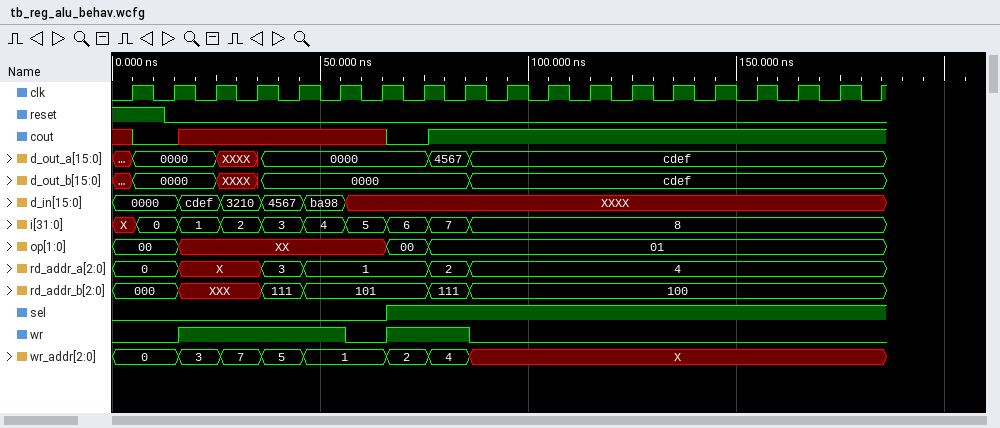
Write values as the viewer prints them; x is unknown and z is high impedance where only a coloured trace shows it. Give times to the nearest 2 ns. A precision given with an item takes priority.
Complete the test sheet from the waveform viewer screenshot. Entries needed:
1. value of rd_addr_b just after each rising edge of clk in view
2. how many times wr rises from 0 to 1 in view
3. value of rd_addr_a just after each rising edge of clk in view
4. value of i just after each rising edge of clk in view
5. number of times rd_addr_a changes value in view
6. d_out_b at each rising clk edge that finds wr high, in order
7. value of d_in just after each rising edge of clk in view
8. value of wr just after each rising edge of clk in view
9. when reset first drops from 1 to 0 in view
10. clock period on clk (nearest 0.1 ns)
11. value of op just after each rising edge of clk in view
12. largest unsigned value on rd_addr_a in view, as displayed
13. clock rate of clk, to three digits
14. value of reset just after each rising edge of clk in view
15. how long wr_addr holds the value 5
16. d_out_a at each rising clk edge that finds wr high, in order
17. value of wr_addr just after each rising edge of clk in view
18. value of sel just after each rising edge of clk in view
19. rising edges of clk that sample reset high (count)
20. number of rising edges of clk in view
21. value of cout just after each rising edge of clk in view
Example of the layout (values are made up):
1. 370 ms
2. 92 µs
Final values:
1. 000, 000, XXX, XXX, 111, 101, 101, 101, 111, 100, 100, 100, 100, 100, 100, 100, 100, 100, 100
2. 2
3. 0, 0, X, X, 3, 1, 1, 1, 2, 4, 4, 4, 4, 4, 4, 4, 4, 4, 4
4. X, 0, 1, 2, 3, 4, 5, 6, 7, 8, 8, 8, 8, 8, 8, 8, 8, 8, 8
5. 5
6. 0000, XXXX, 0000, 0000, 0000, 0000
7. 0000, 0000, cdef, 3210, 4567, ba98, XXXX, XXXX, XXXX, XXXX, XXXX, XXXX, XXXX, XXXX, XXXX, XXXX, XXXX, XXXX, XXXX
8. 0 0 1 1 1 1 0 1 1 0 0 0 0 0 0 0 0 0 0
9. 12 ns
10. 10 ns
11. 00, 00, XX, XX, XX, XX, XX, 00, 01, 01, 01, 01, 01, 01, 01, 01, 01, 01, 01
12. 4
13. 100 MHz
14. 1 0 0 0 0 0 0 0 0 0 0 0 0 0 0 0 0 0 0
15. 10 ns
16. 0000, XXXX, 0000, 0000, 0000, 4567
17. 0, 0, 3, 7, 5, 1, 1, 2, 4, X, X, X, X, X, X, X, X, X, X
18. 0 0 0 0 0 0 0 1 1 1 1 1 1 1 1 1 1 1 1
19. 1
20. 19
21. 0 0 x x x x x 0 1 1 1 1 1 1 1 1 1 1 1
